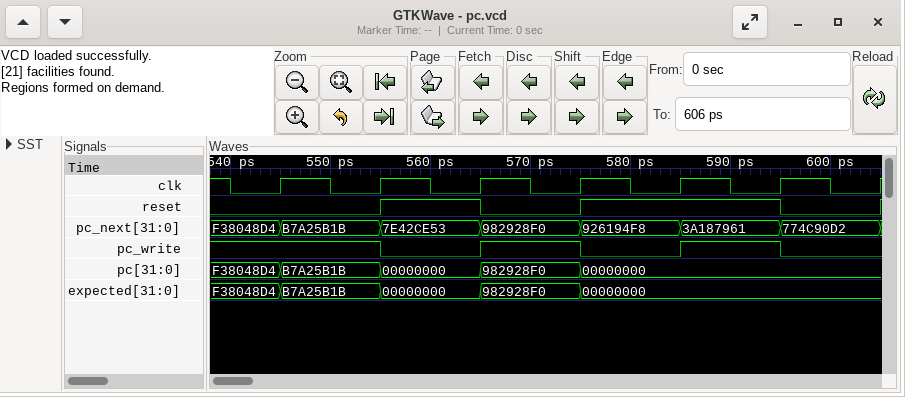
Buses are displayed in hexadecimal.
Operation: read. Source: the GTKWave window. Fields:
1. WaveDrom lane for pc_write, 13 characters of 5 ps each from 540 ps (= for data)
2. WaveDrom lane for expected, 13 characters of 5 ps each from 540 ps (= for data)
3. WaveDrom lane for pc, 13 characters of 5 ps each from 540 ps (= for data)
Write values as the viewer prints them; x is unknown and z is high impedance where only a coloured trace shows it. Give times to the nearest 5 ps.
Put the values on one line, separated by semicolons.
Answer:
{name: 'pc_write', wave: '1..0.1.0.1.0.'}; {name: 'expected', wave: '==.=.=.=.....', data: 'F38048D4 B7A25B1B 00000000 982928F0 00000000'}; {name: 'pc', wave: '==.=.=.=.....', data: 'F38048D4 B7A25B1B 00000000 982928F0 00000000'}
